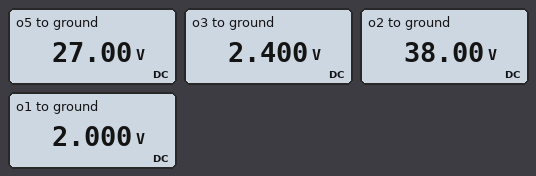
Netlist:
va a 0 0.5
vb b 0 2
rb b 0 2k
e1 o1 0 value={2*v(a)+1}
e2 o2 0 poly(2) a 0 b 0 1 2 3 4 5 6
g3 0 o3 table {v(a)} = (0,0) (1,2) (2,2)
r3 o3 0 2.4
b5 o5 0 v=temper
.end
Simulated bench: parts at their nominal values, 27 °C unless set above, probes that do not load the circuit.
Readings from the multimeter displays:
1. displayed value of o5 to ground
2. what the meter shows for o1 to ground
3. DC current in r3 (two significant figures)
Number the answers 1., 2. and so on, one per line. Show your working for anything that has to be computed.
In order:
1. 27.00 V
2. 2.000 V
3. (2.4 V) / 2.4 Ω = 1.0 A
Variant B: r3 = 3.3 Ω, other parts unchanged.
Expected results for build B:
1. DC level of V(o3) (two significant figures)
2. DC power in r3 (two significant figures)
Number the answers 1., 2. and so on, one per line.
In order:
1. 3.3 V
2. 3.3 W
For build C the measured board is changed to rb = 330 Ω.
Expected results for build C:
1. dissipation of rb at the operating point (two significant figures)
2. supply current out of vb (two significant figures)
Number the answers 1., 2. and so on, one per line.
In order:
1. 12 mW
2. 6.1 mA
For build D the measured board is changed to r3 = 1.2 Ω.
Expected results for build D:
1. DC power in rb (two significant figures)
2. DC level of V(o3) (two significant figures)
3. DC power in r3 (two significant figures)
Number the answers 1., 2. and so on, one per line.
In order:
1. 2.0 mW
2. 1.2 V
3. 1.2 W
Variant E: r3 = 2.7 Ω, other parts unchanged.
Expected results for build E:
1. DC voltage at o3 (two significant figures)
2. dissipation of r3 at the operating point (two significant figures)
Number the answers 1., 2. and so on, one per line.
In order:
1. 2.7 V
2. 2.7 W
